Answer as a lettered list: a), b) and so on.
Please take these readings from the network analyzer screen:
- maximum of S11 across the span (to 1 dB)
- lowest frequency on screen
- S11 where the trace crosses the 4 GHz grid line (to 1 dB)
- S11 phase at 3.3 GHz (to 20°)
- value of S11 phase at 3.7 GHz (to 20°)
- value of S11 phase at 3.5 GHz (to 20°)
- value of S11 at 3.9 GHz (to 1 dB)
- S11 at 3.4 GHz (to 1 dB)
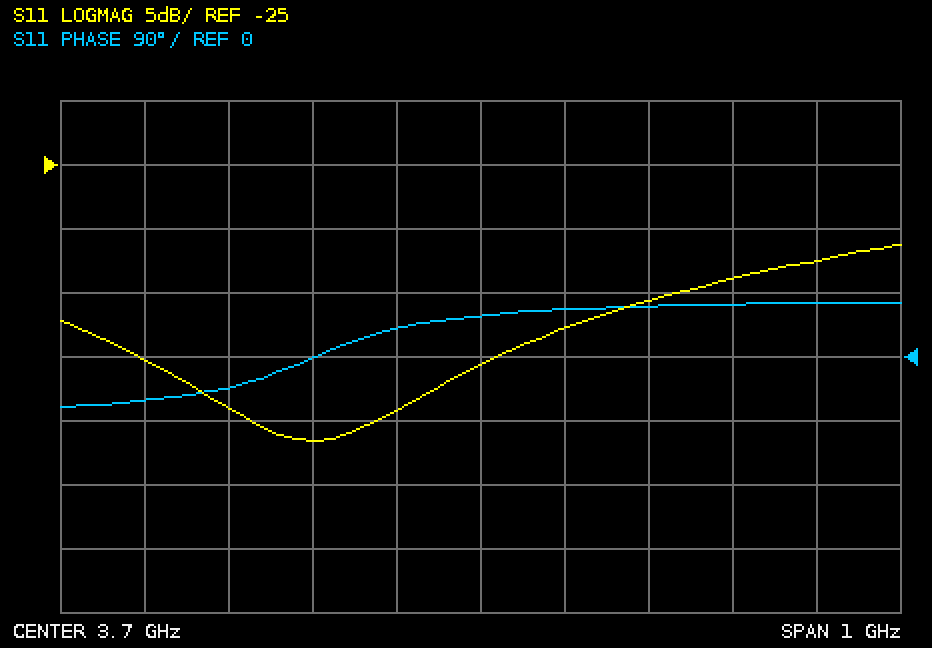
a) -31 dB
b) 3.2 GHz
c) -34 dB
d) -60°
e) 60°
f) 0°
g) -36 dB
h) -44 dB
